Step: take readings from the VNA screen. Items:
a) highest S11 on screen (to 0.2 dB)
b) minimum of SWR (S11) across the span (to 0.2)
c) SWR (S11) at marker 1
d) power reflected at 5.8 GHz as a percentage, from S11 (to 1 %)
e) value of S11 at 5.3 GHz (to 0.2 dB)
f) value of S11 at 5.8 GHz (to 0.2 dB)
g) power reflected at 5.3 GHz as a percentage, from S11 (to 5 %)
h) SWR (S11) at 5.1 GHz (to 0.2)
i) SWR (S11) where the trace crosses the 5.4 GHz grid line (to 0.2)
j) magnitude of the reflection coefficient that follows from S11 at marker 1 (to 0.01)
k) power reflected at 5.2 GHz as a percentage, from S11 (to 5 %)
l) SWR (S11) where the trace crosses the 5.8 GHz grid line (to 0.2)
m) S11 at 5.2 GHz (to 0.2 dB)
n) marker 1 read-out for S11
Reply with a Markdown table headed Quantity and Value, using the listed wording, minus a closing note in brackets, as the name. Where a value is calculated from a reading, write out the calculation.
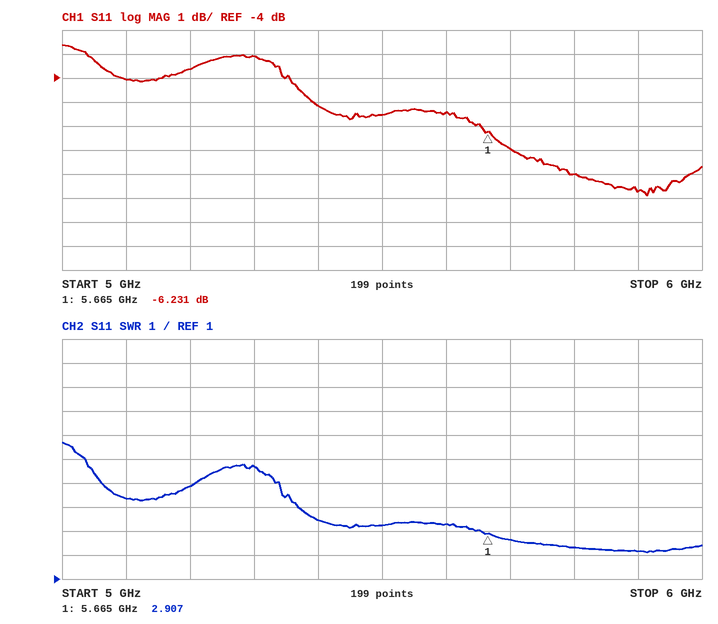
| Quantity | Value |
|---|---|
| highest S11 on screen | -2.6 dB |
| minimum of SWR (S11) across the span | 2.2 |
| SWR (S11) at marker 1 | 2.907 |
| power reflected at 5.8 GHz as a percentage, from S11 | 10^(-8/10) ≈ 16 % |
| value of S11 at 5.3 GHz | -3.0 dB |
| value of S11 at 5.8 GHz | -8.0 dB |
| power reflected at 5.3 GHz as a percentage, from S11 | 10^(-3/10) ≈ 50 % |
| SWR (S11) at 5.1 GHz | 4.4 |
| SWR (S11) where the trace crosses the 5.4 GHz grid line | 3.4 |
| magnitude of the reflection coefficient that follows from S11 at marker 1 | 10^(-6.231/20) ≈ 0.49 |
| power reflected at 5.2 GHz as a percentage, from S11 | 10^(-3.6/10) ≈ 43.7 %, so 45 % to the nearest 5 % |
| SWR (S11) where the trace crosses the 5.8 GHz grid line | 2.4 |
| S11 at 5.2 GHz | -3.6 dB |
| marker 1 read-out for S11 | -6.231 dB |
